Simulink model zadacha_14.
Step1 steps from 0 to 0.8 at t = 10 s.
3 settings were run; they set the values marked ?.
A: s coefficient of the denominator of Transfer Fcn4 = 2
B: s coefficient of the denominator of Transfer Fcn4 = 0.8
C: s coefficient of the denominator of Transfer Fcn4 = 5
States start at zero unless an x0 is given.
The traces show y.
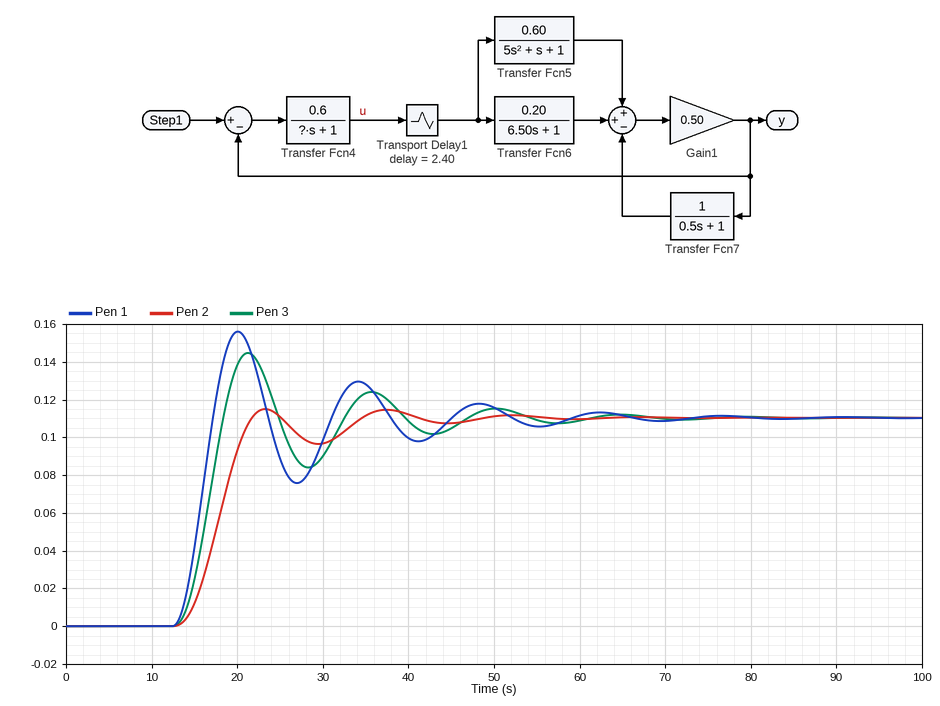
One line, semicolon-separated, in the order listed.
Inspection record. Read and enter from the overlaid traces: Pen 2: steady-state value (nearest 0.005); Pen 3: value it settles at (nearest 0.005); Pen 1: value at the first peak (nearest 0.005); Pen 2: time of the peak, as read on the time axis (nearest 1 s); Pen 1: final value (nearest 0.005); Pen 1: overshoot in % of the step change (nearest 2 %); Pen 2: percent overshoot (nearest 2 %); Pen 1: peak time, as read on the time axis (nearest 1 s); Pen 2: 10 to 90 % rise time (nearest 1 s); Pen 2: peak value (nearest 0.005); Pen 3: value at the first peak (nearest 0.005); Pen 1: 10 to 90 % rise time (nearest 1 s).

0.110; 0.110; 0.155; 23 s; 0.110; 42 %; 4 %; 20 s; 6 s; 0.115; 0.145; 3 s
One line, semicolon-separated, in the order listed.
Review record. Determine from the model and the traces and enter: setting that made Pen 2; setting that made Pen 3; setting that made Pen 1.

C; A; B
